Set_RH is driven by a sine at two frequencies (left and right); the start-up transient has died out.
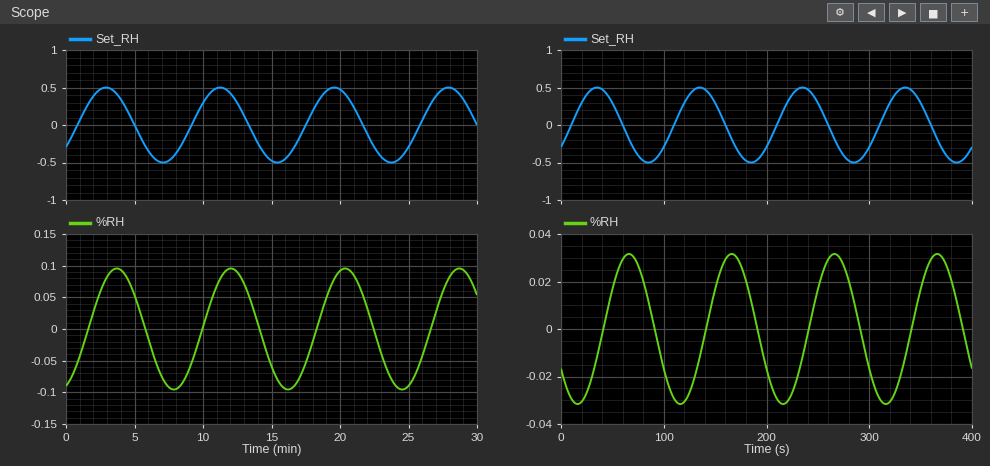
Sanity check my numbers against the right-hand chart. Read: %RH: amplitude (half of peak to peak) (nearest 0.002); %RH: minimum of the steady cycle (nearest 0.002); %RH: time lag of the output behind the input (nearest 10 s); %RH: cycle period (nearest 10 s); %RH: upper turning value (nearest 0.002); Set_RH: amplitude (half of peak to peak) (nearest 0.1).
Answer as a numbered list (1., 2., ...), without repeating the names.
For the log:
1. 0.032
2. -0.032
3. 30 s
4. 100 s
5. 0.032
6. 0.5
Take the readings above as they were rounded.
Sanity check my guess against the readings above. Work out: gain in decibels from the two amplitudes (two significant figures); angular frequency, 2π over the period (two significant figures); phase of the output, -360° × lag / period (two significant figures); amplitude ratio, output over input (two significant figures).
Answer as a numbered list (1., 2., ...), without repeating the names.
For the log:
1. -24 dB
2. 0.063 rad/s
3. -110°
4. 0.064
